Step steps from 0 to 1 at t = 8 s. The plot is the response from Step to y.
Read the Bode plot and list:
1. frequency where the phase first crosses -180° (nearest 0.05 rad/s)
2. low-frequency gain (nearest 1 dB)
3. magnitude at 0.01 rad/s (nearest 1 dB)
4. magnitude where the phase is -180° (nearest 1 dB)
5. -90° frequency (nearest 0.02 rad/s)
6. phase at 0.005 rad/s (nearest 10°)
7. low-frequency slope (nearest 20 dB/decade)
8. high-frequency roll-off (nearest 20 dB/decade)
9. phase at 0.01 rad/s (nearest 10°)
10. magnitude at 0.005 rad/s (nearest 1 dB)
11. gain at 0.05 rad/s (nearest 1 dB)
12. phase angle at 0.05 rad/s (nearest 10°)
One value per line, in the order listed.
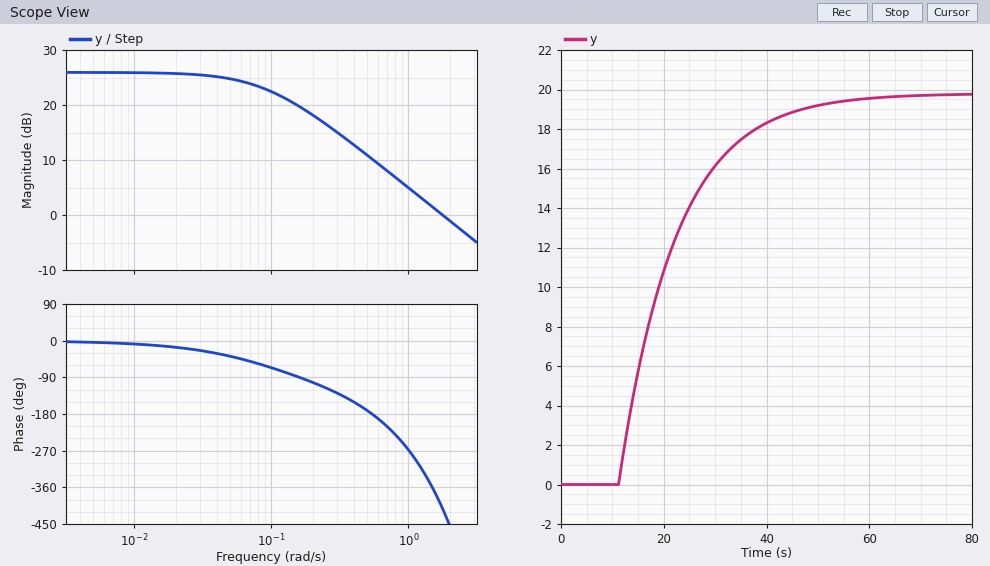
0.55 rad/s
26 dB
26 dB
10 dB
0.16 rad/s
0°
0 dB/decade
-20 dB/decade
-10°
26 dB
25 dB
-40°
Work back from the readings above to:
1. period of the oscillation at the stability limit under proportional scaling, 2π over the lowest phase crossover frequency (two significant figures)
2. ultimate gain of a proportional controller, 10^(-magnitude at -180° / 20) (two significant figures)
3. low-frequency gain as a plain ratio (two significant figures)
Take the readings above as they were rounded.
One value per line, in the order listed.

11 s
0.32
20
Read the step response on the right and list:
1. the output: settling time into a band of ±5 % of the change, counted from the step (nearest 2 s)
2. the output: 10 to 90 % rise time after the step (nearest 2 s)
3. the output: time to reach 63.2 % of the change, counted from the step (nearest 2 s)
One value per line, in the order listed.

36 s
24 s
14 s
